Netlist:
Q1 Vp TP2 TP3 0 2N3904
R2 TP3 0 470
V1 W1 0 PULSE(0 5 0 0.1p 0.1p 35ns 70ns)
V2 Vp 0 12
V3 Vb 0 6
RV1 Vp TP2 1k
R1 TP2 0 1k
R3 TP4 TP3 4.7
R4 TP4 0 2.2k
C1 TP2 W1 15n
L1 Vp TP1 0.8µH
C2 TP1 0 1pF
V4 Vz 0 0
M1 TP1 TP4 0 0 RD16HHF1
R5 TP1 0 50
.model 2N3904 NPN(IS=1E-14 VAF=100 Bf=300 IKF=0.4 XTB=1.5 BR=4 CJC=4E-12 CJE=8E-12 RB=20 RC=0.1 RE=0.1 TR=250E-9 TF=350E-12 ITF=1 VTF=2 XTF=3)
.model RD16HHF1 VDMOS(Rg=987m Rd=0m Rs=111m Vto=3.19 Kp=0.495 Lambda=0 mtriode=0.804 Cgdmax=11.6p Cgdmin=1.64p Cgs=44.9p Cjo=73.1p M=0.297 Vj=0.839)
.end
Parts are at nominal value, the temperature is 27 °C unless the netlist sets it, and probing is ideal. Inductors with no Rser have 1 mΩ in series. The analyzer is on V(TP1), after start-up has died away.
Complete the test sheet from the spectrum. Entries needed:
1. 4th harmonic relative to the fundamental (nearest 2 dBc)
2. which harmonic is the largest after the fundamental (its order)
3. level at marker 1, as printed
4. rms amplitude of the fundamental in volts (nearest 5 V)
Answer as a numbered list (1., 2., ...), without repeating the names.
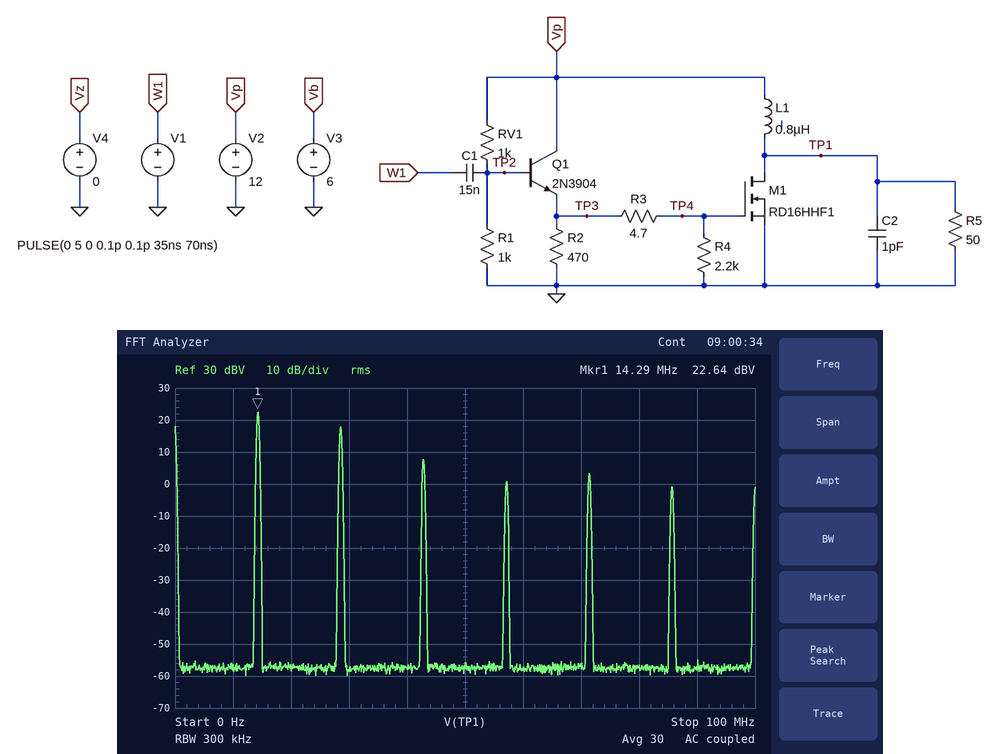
1. -22 dBc
2. 2
3. 22.64 dBV
4. 15 V
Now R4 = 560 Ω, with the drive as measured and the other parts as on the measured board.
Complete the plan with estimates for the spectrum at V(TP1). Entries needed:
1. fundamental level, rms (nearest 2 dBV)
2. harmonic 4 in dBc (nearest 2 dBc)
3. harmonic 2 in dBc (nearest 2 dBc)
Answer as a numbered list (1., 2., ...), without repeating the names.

1. 22 dBV
2. -14 dBc
3. -6 dBc
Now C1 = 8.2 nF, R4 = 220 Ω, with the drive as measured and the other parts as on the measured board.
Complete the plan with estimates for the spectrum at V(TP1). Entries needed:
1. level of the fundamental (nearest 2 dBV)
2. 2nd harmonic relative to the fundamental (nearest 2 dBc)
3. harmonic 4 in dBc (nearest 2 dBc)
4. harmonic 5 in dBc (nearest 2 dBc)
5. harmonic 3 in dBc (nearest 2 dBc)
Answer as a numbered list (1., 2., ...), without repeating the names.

1. 22 dBV
2. -10 dBc
3. -14 dBc
4. -26 dBc
5. -12 dBc
